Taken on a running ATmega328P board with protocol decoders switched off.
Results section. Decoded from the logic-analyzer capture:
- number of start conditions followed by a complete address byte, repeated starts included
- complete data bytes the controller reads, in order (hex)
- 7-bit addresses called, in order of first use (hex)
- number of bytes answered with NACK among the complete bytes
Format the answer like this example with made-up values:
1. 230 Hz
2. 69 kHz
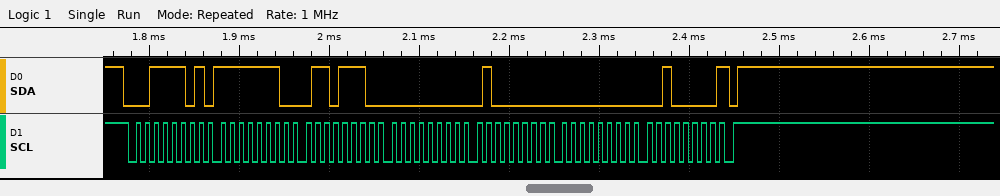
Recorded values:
1. 1
2. FE 6E 00 40 00 20
3. 0x1E
4. 1
